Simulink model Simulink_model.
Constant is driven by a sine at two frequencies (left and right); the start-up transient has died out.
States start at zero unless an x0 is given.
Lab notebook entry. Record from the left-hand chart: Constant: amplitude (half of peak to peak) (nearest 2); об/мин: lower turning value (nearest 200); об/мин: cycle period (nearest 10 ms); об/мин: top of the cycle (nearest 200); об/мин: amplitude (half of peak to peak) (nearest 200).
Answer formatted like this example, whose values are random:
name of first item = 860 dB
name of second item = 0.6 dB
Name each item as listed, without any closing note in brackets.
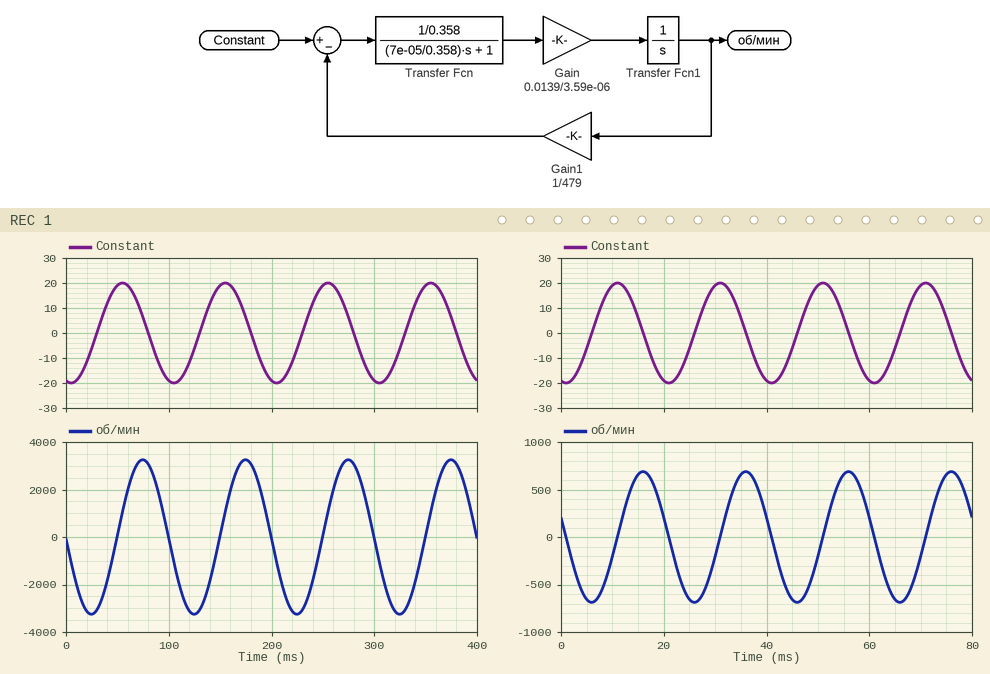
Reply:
Constant: amplitude (half of peak to peak) = 20
об/мин: lower turning value = -3200
об/мин: cycle period = 100 ms
об/мин: top of the cycle = 3200
об/мин: amplitude (half of peak to peak) = 3200
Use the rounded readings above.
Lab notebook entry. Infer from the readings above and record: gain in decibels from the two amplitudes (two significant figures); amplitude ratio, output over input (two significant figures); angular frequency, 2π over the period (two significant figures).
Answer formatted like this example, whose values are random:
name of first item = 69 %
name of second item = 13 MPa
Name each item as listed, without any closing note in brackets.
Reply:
gain in decibels from the two amplitudes = 44 dB
amplitude ratio, output over input = 160
angular frequency, 2π over the period = 0.063 rad/ms
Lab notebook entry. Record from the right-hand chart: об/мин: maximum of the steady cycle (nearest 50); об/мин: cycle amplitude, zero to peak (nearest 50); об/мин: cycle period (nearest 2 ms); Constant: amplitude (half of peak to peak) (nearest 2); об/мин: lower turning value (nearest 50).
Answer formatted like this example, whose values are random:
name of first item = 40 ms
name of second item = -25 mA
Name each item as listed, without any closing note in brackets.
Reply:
об/мин: maximum of the steady cycle = 700
об/мин: cycle amplitude, zero to peak = 700
об/мин: cycle period = 20 ms
Constant: amplitude (half of peak to peak) = 20
об/мин: lower turning value = -700
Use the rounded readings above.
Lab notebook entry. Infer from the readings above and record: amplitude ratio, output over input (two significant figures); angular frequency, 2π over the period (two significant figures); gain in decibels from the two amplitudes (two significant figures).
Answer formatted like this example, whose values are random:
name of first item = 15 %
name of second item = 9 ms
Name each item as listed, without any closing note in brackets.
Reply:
amplitude ratio, output over input = 35
angular frequency, 2π over the period = 0.31 rad/ms
gain in decibels from the two amplitudes = 31 dB
